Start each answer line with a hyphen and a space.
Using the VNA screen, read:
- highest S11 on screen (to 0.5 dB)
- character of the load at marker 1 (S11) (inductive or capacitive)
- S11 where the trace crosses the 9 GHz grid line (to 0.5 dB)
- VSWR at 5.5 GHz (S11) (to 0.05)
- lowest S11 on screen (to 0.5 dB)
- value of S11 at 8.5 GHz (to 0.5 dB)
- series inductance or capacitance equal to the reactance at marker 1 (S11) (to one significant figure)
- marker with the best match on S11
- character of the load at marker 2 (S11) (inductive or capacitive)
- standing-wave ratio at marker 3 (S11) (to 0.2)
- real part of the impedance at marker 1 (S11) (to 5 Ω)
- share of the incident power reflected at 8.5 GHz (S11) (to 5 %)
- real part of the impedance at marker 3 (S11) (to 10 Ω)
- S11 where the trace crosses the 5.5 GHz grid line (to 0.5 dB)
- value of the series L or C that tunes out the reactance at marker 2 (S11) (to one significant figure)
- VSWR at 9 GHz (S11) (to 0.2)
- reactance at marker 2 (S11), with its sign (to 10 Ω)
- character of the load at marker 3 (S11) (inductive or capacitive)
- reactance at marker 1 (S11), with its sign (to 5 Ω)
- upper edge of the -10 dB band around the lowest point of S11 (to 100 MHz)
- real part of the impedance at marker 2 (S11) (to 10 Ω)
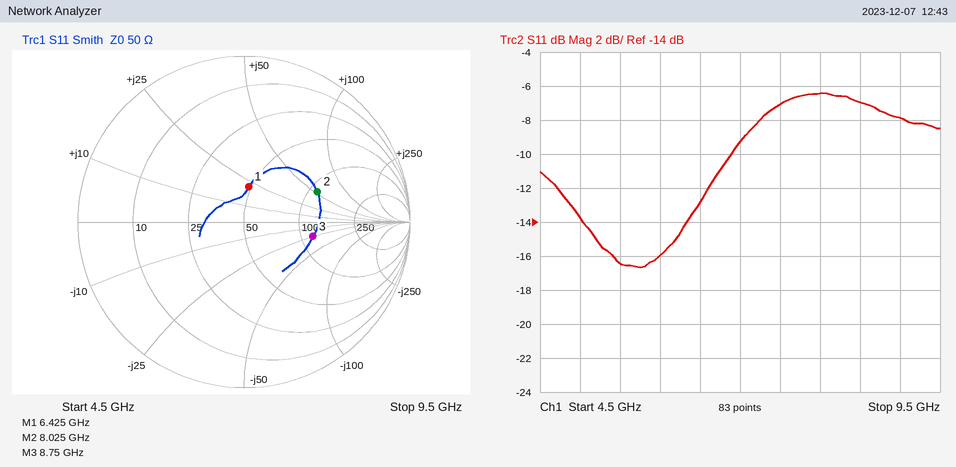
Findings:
- -6.5 dB
- inductive
- -8.0 dB
- 1.35
- -16.5 dB
- -7.0 dB
- 500 pH
- marker 1
- inductive
- 2.4
- 50 Ω
- 20 %
- 120 Ω
- -16.5 dB
- 400 fF
- 2.4
- +50 Ω
- capacitive
- +20 Ω
- 6.9 GHz
- 110 Ω
